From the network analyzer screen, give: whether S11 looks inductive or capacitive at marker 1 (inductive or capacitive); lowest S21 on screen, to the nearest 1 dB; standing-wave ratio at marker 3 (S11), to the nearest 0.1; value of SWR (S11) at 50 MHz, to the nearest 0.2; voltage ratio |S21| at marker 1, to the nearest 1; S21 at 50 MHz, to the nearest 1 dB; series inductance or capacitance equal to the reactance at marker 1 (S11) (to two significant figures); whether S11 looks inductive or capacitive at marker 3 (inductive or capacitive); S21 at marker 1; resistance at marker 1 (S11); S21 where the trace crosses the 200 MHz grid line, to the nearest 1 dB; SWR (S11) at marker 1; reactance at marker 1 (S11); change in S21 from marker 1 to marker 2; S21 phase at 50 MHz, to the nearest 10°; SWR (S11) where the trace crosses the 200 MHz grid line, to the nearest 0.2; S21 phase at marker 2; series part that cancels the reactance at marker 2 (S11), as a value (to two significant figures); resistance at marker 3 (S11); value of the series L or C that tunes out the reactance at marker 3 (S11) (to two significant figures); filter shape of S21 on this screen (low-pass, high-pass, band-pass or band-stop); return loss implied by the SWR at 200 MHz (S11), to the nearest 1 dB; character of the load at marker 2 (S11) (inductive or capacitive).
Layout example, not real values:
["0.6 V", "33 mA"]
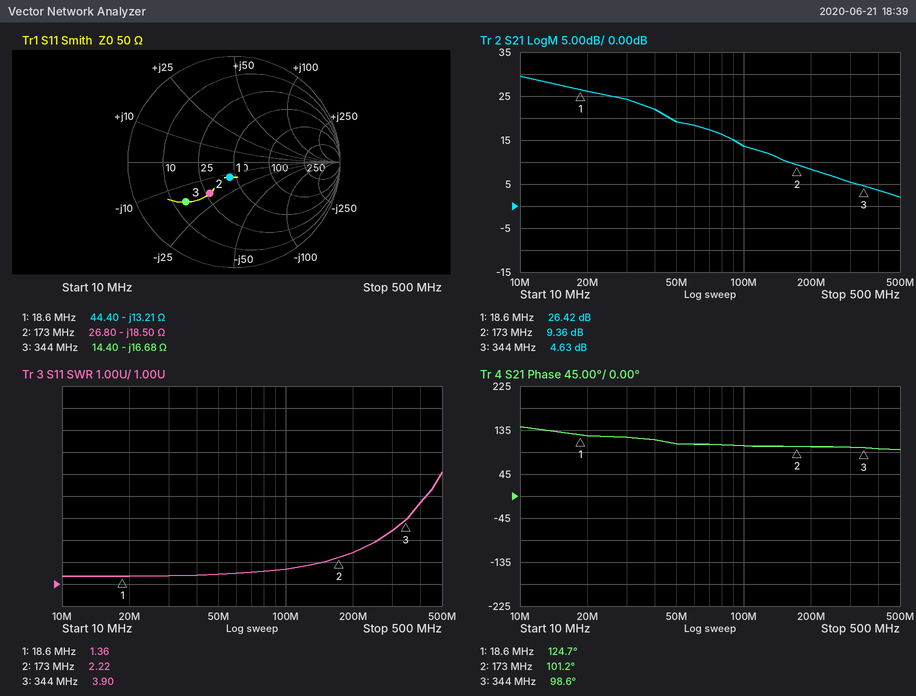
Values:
["capacitive", "2 dB", "3.9", "1.4", "21", "19 dB", "650 pF", "capacitive", "26.42 dB", "44.40 Ω", "8 dB", "1.36", "-13.21 Ω", "-17.06 dB", "110°", "2.4", "101.2°", "17 nH", "14.40 Ω", "7.7 nH", "low-pass", "8 dB", "capacitive"]
